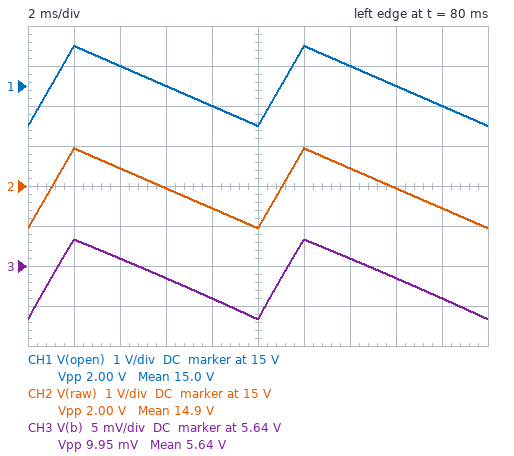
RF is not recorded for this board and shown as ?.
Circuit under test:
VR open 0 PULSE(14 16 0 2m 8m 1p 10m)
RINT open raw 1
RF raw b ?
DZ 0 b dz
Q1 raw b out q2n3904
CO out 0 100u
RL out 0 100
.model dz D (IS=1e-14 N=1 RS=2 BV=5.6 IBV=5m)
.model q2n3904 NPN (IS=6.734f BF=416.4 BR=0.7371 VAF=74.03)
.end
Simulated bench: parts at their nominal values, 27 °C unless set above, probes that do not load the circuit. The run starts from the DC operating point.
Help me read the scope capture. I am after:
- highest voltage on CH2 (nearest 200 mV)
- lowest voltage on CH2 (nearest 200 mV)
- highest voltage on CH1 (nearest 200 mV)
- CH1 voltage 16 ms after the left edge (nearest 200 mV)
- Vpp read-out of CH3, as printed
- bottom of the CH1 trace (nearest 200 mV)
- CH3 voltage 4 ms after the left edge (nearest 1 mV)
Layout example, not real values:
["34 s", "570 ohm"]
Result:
["16.0 V", "14.0 V", "16.0 V", "15.0 V", "9.95 mV", "14.0 V", "5.641 V"]
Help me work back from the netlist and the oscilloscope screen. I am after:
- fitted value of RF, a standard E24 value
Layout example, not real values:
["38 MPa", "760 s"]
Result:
["910 Ω"]
